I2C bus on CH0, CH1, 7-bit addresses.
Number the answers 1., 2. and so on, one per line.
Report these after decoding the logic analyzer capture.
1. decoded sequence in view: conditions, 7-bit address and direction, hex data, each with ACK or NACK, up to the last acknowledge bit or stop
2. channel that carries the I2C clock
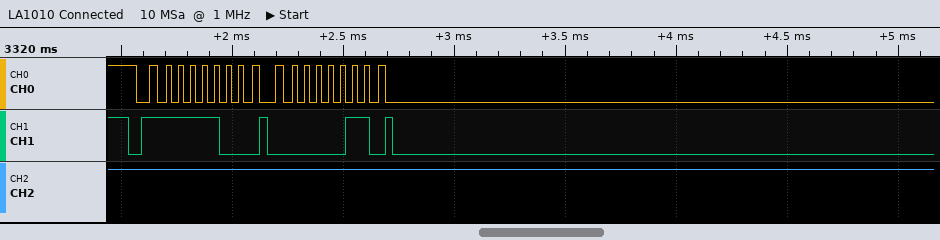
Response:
1. start, address 7E write ACK, 03 ACK
2. CH0
